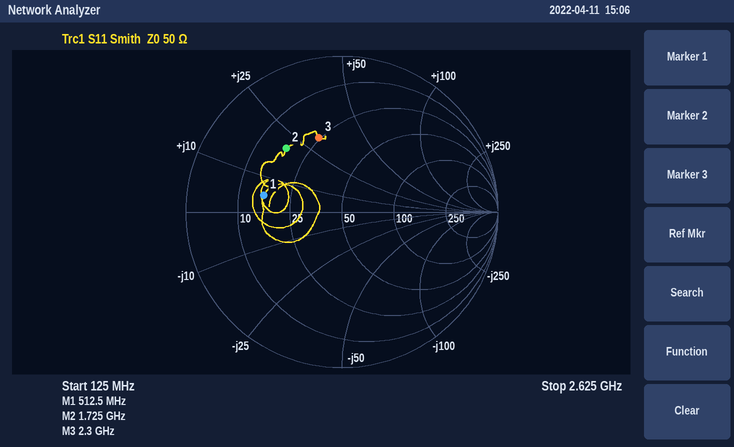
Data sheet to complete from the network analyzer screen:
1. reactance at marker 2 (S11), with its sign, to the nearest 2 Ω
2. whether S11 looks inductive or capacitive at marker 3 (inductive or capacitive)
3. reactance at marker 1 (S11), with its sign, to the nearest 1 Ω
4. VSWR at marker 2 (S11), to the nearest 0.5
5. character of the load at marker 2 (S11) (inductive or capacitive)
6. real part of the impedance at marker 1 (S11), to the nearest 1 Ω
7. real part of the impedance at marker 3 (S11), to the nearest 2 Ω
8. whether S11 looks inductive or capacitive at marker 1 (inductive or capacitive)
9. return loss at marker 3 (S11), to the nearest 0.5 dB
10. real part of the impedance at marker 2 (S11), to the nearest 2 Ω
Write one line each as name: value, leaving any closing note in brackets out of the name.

reactance at marker 2 (S11), with its sign, to the nearest 2 Ω: +20 Ω
whether S11 looks inductive or capacitive at marker 3: inductive
reactance at marker 1 (S11), with its sign, to the nearest 1 Ω: +5 Ω
VSWR at marker 2 (S11), to the nearest 0.5: 3.5
character of the load at marker 2 (S11): inductive
real part of the impedance at marker 1 (S11), to the nearest 1 Ω: 16 Ω
real part of the impedance at marker 3 (S11), to the nearest 2 Ω: 24 Ω
whether S11 looks inductive or capacitive at marker 1: inductive
return loss at marker 3 (S11), to the nearest 0.5 dB: 6.0 dB
real part of the impedance at marker 2 (S11), to the nearest 2 Ω: 18 Ω
